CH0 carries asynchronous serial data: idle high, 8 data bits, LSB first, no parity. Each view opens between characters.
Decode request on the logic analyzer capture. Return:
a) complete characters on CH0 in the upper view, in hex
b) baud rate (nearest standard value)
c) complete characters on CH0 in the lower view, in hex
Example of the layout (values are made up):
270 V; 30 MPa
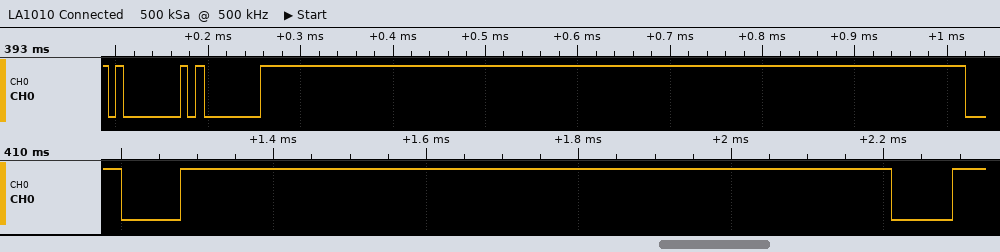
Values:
01, 01; 115200 baud; 00, 00
